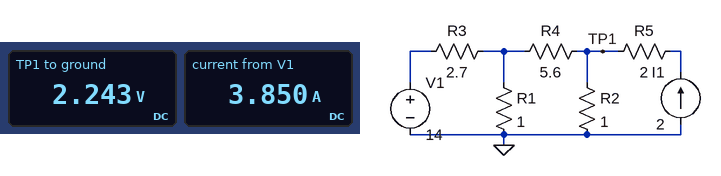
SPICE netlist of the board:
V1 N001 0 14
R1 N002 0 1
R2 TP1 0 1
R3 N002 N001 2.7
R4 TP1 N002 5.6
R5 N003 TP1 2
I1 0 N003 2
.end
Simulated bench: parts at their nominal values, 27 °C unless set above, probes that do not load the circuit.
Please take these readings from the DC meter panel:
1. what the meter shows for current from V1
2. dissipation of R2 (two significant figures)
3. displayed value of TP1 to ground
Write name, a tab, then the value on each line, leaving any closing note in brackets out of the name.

what the meter shows for current from V1	3.850 A
dissipation of R2	5.0 W
displayed value of TP1 to ground	2.243 V
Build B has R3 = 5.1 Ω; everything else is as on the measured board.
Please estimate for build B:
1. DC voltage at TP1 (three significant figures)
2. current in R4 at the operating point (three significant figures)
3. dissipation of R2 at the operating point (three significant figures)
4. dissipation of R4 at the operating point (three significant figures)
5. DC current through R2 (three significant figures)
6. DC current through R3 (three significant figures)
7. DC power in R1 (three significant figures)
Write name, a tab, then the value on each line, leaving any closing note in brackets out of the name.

DC voltage at TP1	2.04 V
current in R4 at the operating point	39.7 mA
dissipation of R2 at the operating point	4.16 W
dissipation of R4 at the operating point	8.82 mW
DC current through R2	2.04 A
DC current through R3	2.30 A
DC power in R1	5.12 W
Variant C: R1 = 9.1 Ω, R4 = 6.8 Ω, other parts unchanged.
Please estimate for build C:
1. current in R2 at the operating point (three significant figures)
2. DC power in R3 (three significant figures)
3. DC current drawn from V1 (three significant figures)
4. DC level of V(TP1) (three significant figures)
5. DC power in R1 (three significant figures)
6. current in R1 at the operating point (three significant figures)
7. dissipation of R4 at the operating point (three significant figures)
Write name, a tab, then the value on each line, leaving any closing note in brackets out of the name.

current in R2 at the operating point	2.89 A
DC power in R3	9.47 W
DC current drawn from V1	1.87 A
DC level of V(TP1)	2.89 V
DC power in R1	8.79 W
current in R1 at the operating point	983 mA
dissipation of R4 at the operating point	5.39 W
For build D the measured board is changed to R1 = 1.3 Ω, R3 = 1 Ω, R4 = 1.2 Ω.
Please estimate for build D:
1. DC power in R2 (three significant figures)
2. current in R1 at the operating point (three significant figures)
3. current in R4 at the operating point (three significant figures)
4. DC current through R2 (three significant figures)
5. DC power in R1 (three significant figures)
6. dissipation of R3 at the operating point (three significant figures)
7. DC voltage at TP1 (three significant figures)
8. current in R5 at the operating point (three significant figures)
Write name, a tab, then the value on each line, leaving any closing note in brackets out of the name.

DC power in R2	17.1 W
current in R1 at the operating point	5.16 A
current in R4 at the operating point	2.14 A
DC current through R2	4.14 A
DC power in R1	34.6 W
dissipation of R3 at the operating point	53.2 W
DC voltage at TP1	4.14 V
current in R5 at the operating point	2.00 A
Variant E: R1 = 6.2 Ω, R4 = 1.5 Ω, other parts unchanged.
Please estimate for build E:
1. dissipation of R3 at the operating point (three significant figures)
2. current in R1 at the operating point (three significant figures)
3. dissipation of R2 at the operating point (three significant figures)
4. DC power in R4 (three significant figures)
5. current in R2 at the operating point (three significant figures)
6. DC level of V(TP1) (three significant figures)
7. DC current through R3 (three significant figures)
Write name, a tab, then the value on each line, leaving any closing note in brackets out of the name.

dissipation of R3 at the operating point	21.3 W
current in R1 at the operating point	1.04 A
dissipation of R2 at the operating point	14.2 W
DC power in R4	4.70 W
current in R2 at the operating point	3.77 A
DC level of V(TP1)	3.77 V
DC current through R3	2.81 A
